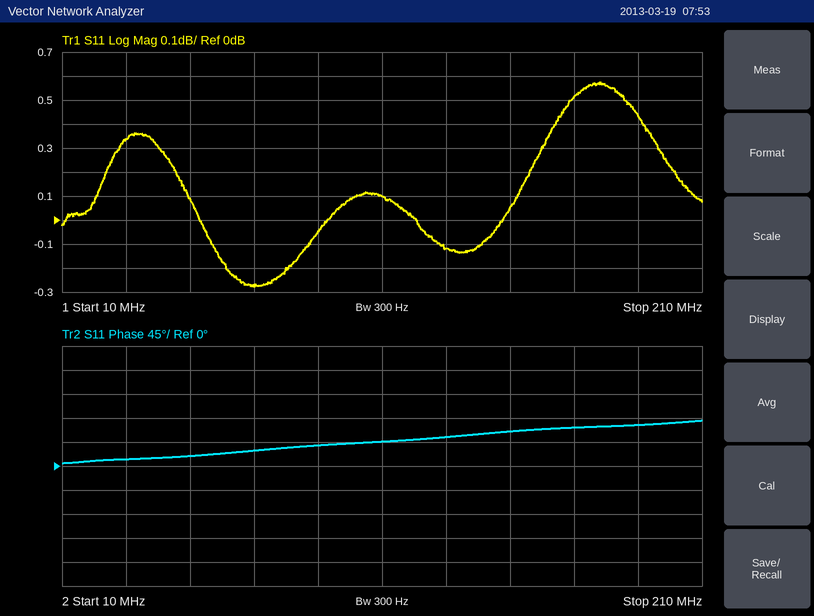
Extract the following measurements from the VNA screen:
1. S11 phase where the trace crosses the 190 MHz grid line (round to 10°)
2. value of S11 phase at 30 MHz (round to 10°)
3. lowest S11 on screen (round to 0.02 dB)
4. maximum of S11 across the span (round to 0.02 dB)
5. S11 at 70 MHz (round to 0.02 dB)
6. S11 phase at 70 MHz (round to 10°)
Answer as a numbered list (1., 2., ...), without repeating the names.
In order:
1. 80°
2. 10°
3. -0.28 dB
4. 0.58 dB
5. -0.28 dB
6. 30°
